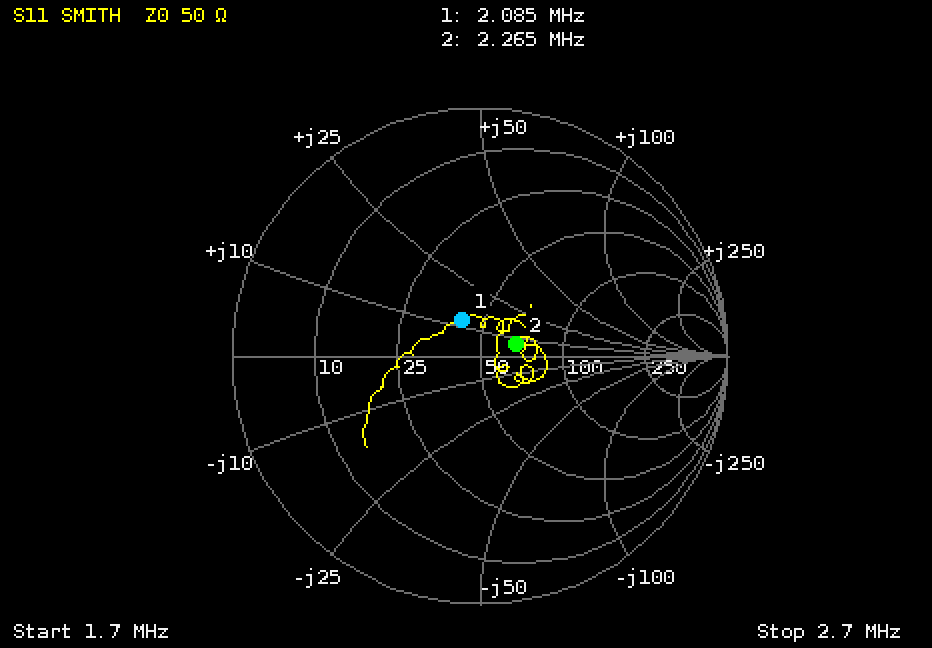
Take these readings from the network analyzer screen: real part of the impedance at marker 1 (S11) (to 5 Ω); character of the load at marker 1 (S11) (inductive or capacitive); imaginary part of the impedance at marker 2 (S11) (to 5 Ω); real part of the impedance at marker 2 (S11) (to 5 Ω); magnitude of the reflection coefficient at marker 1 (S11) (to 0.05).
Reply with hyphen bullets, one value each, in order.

- 40 Ω
- inductive
- +5 Ω
- 65 Ω
- 0.15
